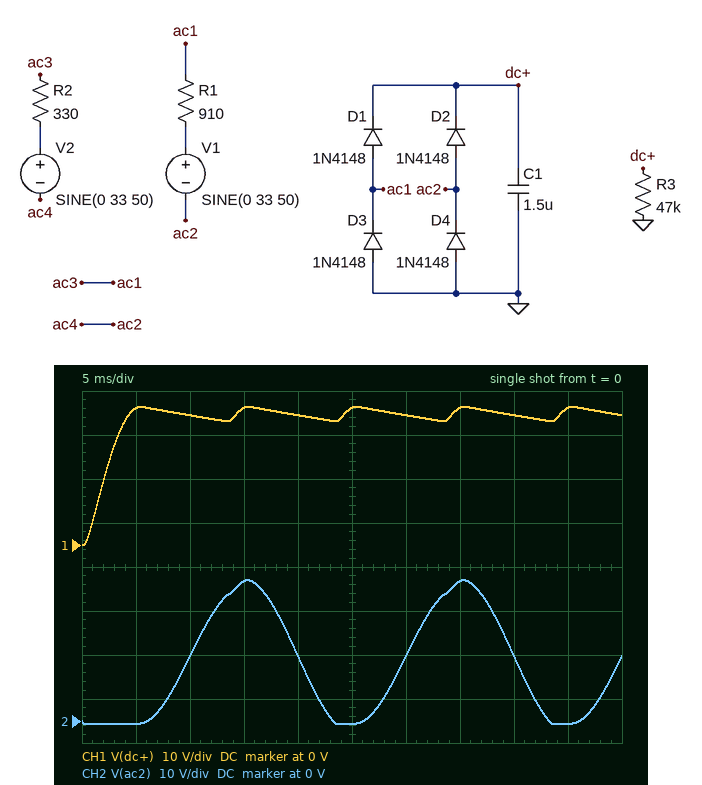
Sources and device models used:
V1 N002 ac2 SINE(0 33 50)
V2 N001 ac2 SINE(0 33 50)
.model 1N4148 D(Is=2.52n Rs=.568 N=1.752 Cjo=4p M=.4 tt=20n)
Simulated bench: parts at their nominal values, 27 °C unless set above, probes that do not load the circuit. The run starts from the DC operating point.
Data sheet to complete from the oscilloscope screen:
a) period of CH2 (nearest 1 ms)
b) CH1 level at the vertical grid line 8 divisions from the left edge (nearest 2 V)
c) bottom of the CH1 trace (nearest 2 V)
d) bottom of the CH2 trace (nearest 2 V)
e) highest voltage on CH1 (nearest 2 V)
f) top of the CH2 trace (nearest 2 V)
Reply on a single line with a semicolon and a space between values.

20 ms; 30 V; 0 V; 0 V; 32 V; 32 V
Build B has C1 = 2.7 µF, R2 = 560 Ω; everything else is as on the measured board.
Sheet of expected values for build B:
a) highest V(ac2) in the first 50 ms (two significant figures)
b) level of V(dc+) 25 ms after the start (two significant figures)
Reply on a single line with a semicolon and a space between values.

31 V; 30 V
